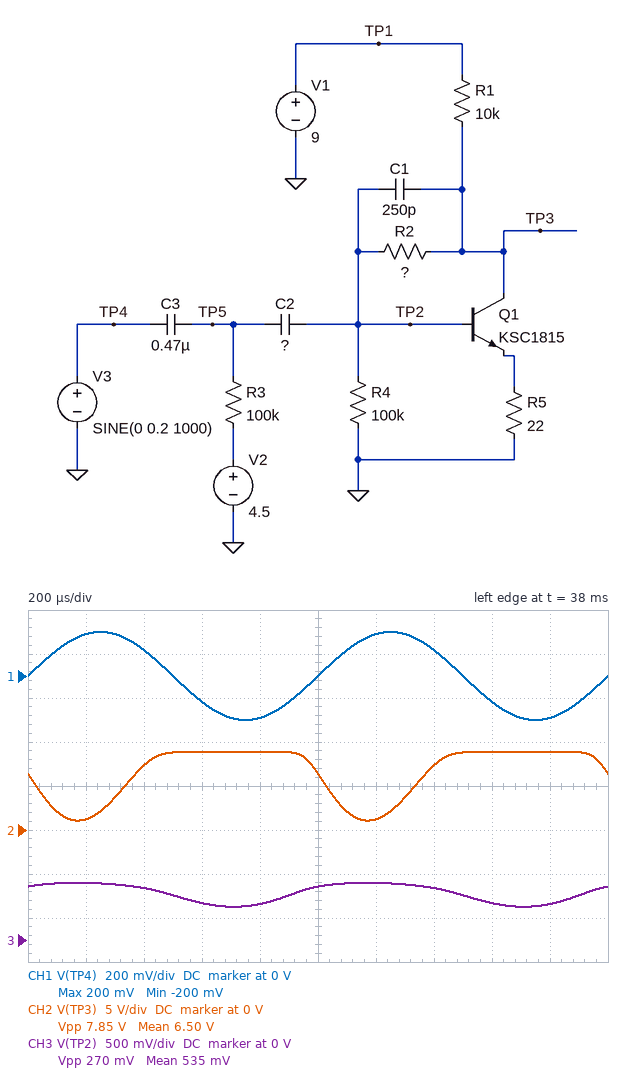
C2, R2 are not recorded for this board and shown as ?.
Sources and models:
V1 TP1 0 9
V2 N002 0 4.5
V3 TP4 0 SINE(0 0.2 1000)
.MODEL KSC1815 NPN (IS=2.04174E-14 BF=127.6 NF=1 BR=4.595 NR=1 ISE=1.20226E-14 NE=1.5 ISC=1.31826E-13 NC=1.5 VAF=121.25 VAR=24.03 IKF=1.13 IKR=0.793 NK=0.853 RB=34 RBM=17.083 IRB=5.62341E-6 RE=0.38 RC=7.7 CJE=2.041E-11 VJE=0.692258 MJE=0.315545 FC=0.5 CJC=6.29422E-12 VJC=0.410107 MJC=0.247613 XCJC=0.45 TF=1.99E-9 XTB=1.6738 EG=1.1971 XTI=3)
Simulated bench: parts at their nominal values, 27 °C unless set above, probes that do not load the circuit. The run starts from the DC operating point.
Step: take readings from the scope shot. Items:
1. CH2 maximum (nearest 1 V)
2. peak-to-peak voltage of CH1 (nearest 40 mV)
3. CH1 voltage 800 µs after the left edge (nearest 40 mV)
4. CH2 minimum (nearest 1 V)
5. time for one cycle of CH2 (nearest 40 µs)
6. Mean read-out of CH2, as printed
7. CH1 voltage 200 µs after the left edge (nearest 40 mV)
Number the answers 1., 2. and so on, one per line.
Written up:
1. 9 V
2. 400 mV
3. -200 mV
4. 1 V
5. 1.00 ms
6. 6.50 V
7. 200 mV
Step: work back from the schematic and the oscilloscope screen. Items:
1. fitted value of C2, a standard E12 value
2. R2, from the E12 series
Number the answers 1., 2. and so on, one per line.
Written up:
1. 22 nF
2. 820 kΩ
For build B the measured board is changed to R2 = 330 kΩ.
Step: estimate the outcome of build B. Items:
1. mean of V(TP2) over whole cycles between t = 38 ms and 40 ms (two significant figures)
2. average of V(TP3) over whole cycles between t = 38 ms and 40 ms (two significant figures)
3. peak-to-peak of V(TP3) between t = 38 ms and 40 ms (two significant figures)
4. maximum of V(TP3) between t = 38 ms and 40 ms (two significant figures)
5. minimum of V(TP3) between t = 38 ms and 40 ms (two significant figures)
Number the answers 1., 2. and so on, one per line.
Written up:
1. 610 mV
2. 4.3 V
3. 8.4 V
4. 8.5 V
5. 110 mV
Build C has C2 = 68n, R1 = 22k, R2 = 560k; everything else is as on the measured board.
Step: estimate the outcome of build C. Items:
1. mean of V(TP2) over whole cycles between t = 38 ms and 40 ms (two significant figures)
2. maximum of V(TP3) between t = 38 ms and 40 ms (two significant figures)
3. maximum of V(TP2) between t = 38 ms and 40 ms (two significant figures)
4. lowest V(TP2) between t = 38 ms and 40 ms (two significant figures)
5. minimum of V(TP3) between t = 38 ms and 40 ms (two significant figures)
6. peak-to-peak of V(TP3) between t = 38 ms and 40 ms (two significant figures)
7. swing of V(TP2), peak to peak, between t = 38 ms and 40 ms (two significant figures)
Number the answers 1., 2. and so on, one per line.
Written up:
1. 490 mV
2. 8.7 V
3. 640 mV
4. 310 mV
5. 46 mV
6. 8.6 V
7. 320 mV
